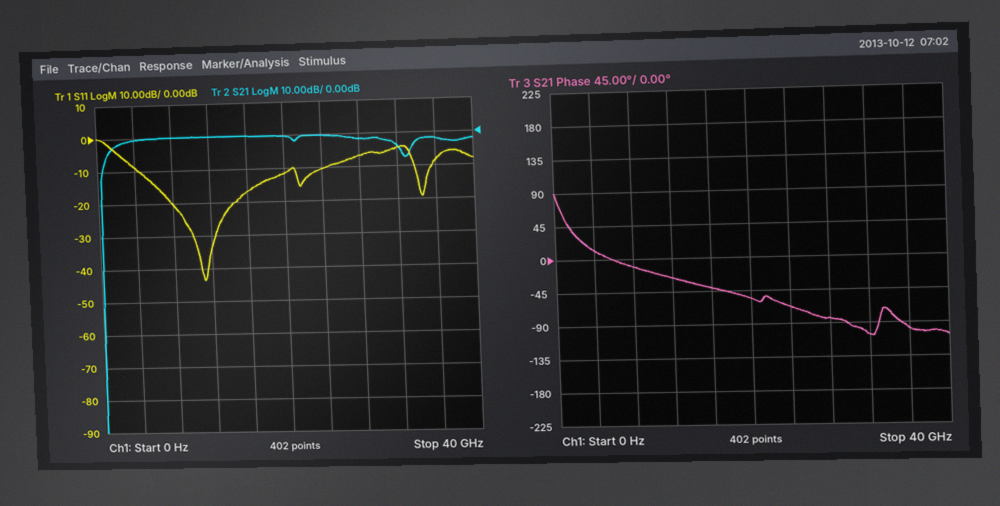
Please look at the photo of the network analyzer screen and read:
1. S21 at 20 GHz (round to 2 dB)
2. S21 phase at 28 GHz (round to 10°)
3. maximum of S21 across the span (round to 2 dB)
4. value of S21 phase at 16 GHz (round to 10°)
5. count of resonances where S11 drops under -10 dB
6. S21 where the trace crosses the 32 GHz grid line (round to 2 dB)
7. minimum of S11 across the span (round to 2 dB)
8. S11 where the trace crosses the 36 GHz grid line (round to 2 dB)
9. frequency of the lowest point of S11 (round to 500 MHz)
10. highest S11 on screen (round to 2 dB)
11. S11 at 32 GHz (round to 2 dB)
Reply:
0 dB
-80°
0 dB
-40°
3
-4 dB
-44 dB
-8 dB
11.0 GHz
0 dB
-4 dB
